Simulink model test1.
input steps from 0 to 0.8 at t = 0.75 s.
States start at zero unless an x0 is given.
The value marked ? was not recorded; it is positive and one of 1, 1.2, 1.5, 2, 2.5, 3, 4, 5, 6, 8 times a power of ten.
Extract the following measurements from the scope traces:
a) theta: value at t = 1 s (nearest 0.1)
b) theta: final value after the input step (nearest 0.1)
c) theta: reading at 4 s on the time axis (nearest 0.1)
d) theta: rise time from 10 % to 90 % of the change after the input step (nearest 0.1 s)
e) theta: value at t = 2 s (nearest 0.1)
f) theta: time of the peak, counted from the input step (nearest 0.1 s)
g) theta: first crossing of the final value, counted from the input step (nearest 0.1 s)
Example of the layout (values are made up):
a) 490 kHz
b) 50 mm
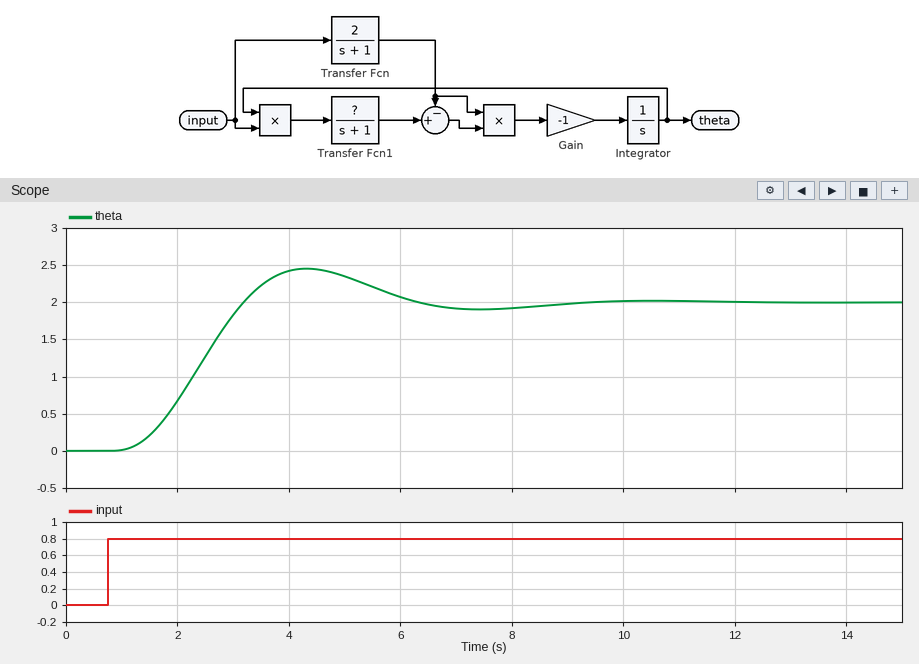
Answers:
a) 0.0
b) 2.0
c) 2.4
d) 1.5 s
e) 0.7
f) 3.6 s
g) 2.4 s
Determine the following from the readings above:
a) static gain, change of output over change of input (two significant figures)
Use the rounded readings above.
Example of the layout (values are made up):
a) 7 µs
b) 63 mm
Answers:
a) 2.5
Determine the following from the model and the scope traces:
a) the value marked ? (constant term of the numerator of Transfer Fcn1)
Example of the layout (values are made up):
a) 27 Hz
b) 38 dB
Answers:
a) 1
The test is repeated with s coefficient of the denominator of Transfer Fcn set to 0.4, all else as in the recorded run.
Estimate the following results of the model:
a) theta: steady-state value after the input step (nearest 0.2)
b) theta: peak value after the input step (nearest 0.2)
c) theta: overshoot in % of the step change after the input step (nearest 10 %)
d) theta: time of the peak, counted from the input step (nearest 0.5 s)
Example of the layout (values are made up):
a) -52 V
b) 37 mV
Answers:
a) 2.0
b) 2.8
c) 40 %
d) 2.5 s
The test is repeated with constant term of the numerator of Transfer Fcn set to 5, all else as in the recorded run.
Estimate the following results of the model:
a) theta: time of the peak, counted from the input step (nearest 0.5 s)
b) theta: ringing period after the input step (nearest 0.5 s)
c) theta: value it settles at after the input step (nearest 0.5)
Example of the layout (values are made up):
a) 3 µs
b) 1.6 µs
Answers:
a) 2.5 s
b) 3.5 s
c) 5.0
